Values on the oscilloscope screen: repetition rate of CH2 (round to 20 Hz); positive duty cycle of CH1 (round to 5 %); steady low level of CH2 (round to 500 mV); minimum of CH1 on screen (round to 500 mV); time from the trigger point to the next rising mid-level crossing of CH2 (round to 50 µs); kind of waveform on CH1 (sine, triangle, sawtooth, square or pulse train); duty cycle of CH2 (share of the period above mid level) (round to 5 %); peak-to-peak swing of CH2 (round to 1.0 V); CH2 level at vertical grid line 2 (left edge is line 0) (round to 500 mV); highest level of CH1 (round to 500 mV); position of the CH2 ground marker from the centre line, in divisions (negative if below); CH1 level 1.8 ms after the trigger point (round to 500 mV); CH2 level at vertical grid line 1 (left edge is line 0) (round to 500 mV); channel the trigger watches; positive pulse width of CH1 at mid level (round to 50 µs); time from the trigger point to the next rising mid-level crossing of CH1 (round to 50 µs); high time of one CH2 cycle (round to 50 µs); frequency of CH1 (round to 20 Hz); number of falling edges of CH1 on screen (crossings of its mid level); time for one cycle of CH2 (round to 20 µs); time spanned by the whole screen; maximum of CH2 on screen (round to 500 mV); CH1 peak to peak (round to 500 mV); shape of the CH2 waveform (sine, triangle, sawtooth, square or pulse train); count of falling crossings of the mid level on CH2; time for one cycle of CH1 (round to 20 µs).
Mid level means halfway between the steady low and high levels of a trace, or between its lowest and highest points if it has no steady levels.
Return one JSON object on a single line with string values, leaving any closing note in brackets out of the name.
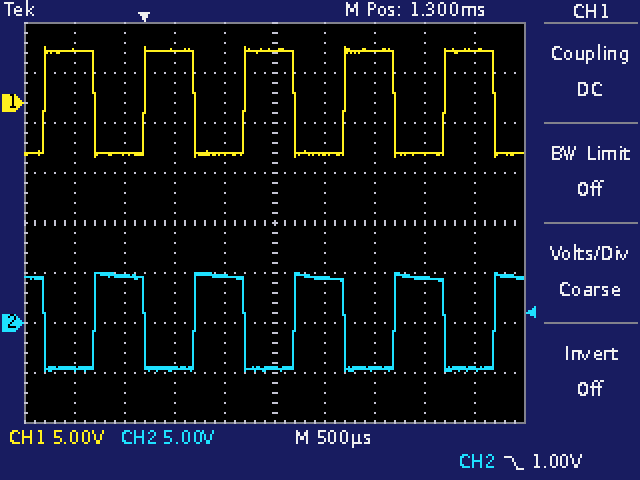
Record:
{"repetition rate of CH2": "1.00 kHz", "positive duty cycle of CH1": "50 %", "steady low level of CH2": "-4.5 V", "minimum of CH1 on screen": "-5.5 V", "time from the trigger point to the next rising mid-level crossing of CH2": "500 µs", "kind of waveform on CH1": "square", "duty cycle of CH2 (share of the period above mid level)": "50 %", "peak-to-peak swing of CH2": "10.0 V", "CH2 level at vertical grid line 2 (left edge is line 0)": "4.5 V", "highest level of CH1": "5.5 V", "position of the CH2 ground marker from the centre line, in divisions": "-2.0 div", "CH1 level 1.8 ms after the trigger point": "-5.0 V", "CH2 level at vertical grid line 1 (left edge is line 0)": "-4.5 V", "channel the trigger watches": "CH2", "positive pulse width of CH1 at mid level": "500 µs", "time from the trigger point to the next rising mid-level crossing of CH1": "1.00 ms", "high time of one CH2 cycle": "500 µs", "frequency of CH1": "1.00 kHz", "number of falling edges of CH1 on screen": "5", "time for one cycle of CH2": "1.00 ms", "time spanned by the whole screen": "5 ms", "maximum of CH2 on screen": "5.0 V", "CH1 peak to peak": "11.0 V", "shape of the CH2 waveform": "square", "count of falling crossings of the mid level on CH2": "5", "time for one cycle of CH1": "1.00 ms"}
